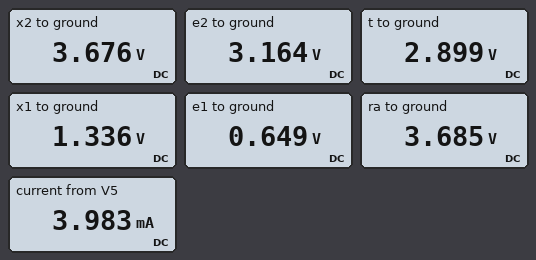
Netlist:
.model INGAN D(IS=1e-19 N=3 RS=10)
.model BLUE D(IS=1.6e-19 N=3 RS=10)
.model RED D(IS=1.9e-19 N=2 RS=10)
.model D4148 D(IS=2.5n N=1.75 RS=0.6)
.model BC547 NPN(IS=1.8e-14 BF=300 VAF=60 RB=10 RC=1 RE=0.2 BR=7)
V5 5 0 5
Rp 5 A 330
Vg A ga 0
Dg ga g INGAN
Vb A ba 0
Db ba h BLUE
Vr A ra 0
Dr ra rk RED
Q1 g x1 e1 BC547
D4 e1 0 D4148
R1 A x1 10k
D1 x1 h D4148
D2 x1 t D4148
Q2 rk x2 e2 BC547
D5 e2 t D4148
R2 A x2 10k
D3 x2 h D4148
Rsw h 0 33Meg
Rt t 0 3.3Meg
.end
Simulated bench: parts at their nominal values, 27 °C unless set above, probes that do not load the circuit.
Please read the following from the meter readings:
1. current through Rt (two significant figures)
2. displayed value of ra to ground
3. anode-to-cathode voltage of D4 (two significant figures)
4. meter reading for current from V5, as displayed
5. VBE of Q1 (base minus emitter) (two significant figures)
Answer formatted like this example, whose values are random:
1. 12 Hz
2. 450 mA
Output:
1. 880 nA
2. 3.685 V
3. 650 mV
4. 3.983 mA
5. 690 mV
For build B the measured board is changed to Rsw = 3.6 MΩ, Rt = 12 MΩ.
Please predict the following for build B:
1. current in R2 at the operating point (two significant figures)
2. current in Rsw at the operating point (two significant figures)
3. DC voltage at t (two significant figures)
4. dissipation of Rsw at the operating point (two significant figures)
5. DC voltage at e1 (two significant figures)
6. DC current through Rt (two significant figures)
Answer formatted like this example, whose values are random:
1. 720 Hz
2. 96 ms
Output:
1. 1.2 µA
2. 950 nA
3. 3.0 V
4. 3.2 µW
5. 650 mV
6. 250 nA
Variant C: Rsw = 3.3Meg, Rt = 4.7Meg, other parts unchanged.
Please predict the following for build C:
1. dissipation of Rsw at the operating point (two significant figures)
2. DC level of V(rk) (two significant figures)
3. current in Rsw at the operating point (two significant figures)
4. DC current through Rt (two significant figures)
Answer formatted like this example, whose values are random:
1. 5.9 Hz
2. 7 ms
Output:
1. 3.5 µW
2. 3.2 V
3. 1.0 µA
4. 620 nA
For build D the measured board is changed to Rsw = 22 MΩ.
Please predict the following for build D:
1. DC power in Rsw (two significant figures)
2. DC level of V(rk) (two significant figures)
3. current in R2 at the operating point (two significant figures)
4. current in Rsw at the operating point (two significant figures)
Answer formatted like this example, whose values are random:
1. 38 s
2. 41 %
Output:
1. 550 nW
2. 3.2 V
3. 1.0 µA
4. 160 nA
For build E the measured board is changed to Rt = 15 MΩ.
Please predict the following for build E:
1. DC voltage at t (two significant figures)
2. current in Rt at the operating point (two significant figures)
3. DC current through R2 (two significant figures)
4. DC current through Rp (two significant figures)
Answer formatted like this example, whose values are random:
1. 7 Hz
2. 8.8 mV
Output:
1. 3.0 V
2. 200 nA
3. 310 nA
4. 4.0 mA
